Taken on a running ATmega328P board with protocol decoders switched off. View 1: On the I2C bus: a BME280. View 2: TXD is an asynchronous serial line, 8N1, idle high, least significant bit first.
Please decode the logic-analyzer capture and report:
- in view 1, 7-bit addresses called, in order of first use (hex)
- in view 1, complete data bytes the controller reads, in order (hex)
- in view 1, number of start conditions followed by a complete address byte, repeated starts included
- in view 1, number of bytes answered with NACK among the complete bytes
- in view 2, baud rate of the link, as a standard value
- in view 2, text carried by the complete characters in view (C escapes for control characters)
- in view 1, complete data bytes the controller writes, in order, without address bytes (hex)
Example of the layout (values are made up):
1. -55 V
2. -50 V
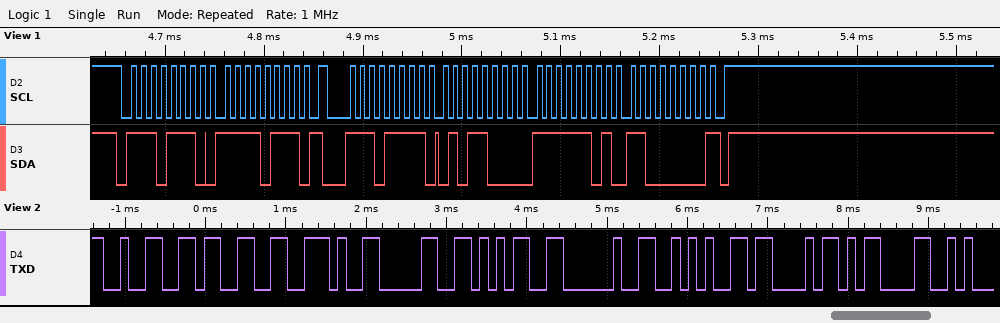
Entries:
1. 0x77
2. 58 FD C0
3. 2
4. 1
5. 9600 baud
6. "23.05 *C\r"
7. F7
